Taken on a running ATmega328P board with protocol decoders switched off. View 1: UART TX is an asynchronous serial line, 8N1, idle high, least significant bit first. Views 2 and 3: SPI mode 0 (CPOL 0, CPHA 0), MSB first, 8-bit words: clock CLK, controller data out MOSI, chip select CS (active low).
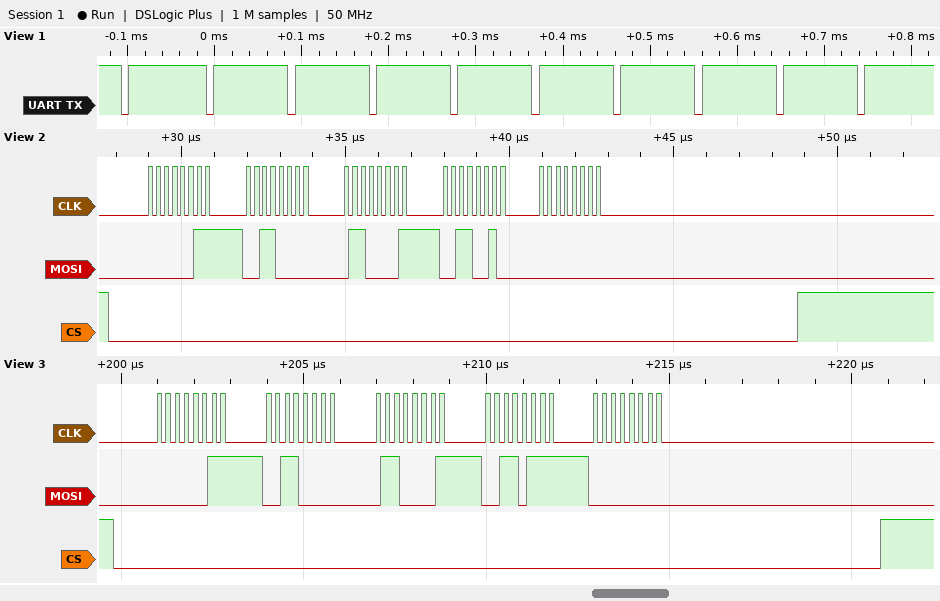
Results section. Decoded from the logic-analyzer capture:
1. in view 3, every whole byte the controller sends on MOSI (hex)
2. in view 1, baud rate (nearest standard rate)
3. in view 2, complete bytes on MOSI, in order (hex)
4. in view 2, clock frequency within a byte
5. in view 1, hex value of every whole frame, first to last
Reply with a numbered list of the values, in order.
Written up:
1. 0x03 0x30 0x61 0x37 0x00
2. 115200 baud
3. 03 30 61 32 00
4. 4 MHz
5. FF FF FF FF FF FF FF FF FF FF
